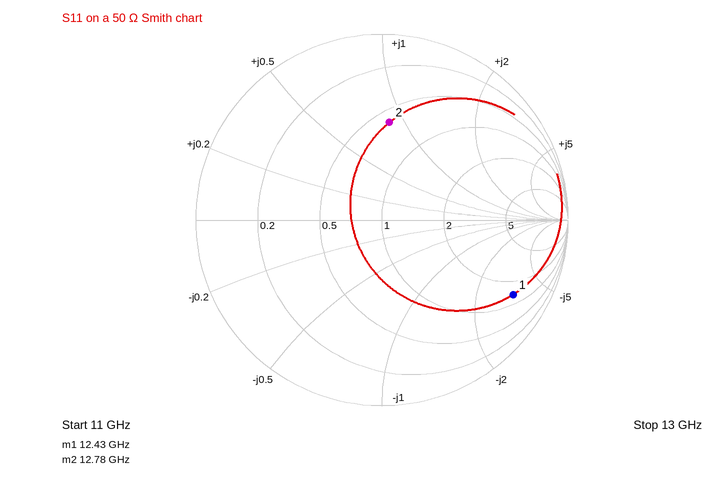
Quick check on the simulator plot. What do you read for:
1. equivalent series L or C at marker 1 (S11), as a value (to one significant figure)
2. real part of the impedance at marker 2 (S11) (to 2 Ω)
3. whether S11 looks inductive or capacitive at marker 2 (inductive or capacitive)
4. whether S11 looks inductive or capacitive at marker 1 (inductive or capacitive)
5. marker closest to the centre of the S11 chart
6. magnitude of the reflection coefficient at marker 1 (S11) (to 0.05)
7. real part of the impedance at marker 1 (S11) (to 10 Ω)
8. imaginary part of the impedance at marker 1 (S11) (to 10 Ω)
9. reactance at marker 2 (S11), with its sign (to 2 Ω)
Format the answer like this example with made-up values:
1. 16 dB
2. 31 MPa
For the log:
1. 80 fF
2. 30 Ω
3. inductive
4. capacitive
5. marker 2
6. 0.80
7. 70 Ω
8. -160 Ω
9. +44 Ω
